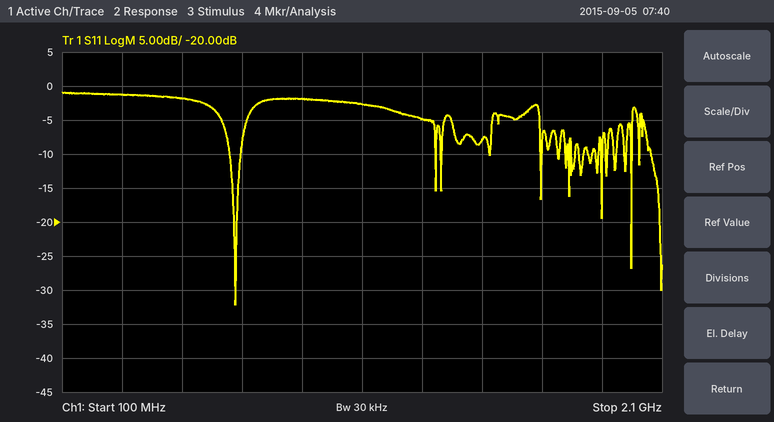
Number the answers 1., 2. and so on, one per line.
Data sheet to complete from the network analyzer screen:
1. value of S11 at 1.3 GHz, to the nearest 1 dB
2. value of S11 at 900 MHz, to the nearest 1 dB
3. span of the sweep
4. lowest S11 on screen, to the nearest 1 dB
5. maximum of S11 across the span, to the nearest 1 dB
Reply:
1. -5 dB
2. -2 dB
3. 2 GHz
4. -32 dB
5. -1 dB
